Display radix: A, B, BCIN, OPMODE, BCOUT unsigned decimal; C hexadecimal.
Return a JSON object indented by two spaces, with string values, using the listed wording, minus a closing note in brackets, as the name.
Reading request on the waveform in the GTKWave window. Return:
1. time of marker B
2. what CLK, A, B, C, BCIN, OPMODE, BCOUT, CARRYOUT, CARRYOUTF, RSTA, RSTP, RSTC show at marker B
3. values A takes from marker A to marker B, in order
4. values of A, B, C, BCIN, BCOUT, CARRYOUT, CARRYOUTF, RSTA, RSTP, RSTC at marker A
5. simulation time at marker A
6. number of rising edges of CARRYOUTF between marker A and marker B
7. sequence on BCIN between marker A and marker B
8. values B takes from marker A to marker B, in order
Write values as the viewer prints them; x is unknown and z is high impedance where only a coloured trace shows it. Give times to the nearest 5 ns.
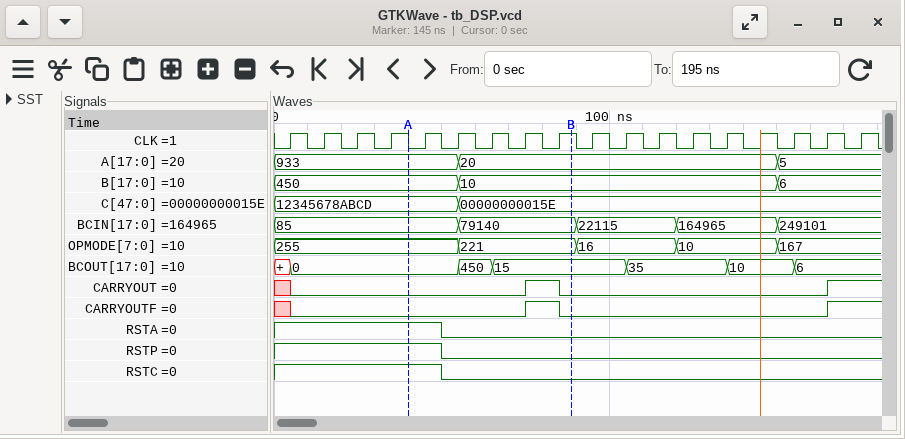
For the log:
{
  "time of marker B": "90 ns",
  "what CLK, A, B, C, BCIN, OPMODE, BCOUT, CARRYOUT, CARRYOUTF, RSTA, RSTP, RSTC show at marker B": "CLK=1, A=20, B=10, C=00000000015E, BCIN=79140, OPMODE=221, BCOUT=15, CARRYOUT=0, CARRYOUTF=0, RSTA=0, RSTP=0, RSTC=0",
  "values A takes from marker A to marker B, in order": "933, 20",
  "values of A, B, C, BCIN, BCOUT, CARRYOUT, CARRYOUTF, RSTA, RSTP, RSTC at marker A": "A=933, B=450, C=12345678ABCD, BCIN=85, BCOUT=0, CARRYOUT=0, CARRYOUTF=0, RSTA=1, RSTP=1, RSTC=1",
  "simulation time at marker A": "40 ns",
  "number of rising edges of CARRYOUTF between marker A and marker B": "1",
  "sequence on BCIN between marker A and marker B": "85, 79140",
  "values B takes from marker A to marker B, in order": "450, 10"
}
